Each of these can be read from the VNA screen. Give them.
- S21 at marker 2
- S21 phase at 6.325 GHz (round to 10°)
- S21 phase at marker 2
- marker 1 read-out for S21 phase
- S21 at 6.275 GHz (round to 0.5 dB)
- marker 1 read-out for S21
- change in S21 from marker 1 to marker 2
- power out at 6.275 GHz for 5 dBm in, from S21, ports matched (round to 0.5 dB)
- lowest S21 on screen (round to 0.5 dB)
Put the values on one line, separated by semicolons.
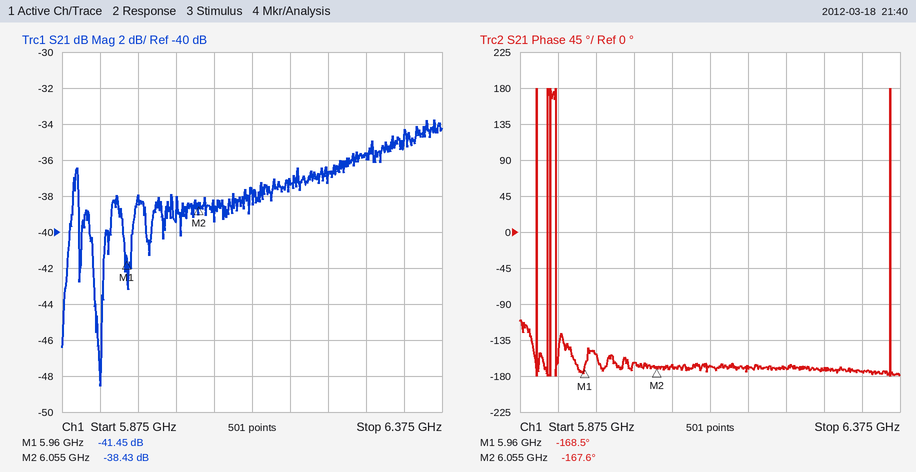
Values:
-38.43 dB; -170°; -167.6°; -168.5°; -35.5 dB; -41.45 dB; 3.02 dB; -30.5 dBm; -48.5 dB
